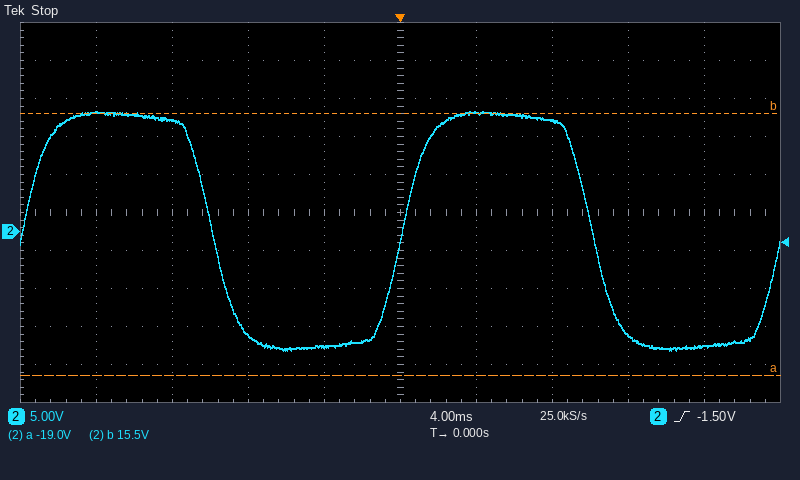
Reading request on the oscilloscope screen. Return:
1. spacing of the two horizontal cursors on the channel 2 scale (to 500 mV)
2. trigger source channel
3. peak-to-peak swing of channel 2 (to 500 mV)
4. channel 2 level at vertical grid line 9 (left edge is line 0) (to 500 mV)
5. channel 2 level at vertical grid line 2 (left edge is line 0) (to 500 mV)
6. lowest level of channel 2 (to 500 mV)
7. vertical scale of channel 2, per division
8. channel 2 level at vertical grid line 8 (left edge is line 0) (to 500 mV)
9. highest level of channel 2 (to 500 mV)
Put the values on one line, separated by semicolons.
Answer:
34.5 V; channel 2; 31.5 V; -15.0 V; 14.5 V; -15.5 V; 5 V; -13.5 V; 16.0 V
